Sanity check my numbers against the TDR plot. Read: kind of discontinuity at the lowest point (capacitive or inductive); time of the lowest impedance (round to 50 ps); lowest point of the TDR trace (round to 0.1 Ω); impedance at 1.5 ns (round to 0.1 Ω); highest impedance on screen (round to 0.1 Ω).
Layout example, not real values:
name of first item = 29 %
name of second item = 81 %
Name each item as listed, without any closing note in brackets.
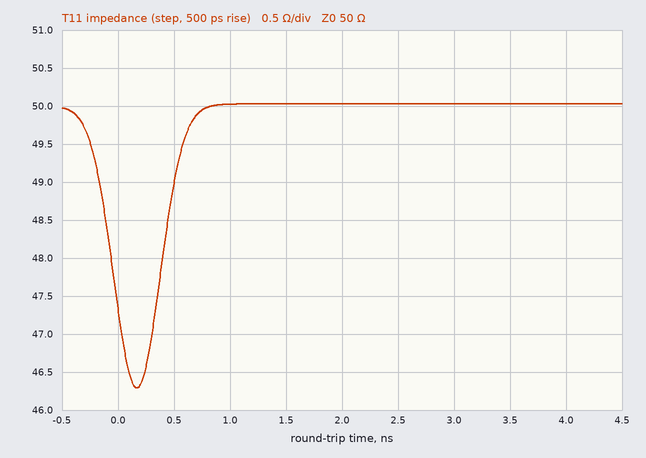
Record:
kind of discontinuity at the lowest point = capacitive
time of the lowest impedance = 150 ps
lowest point of the TDR trace = 46.3 Ω
impedance at 1.5 ns = 50.0 Ω
highest impedance on screen = 50.0 Ω
